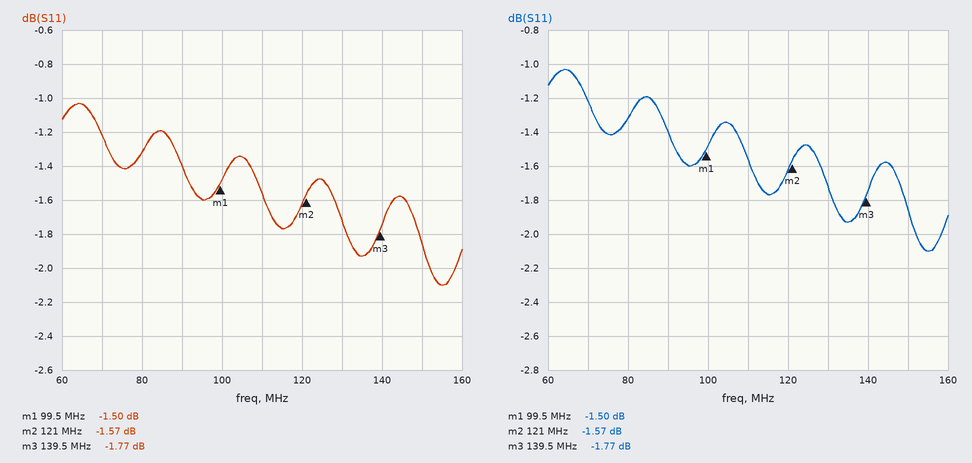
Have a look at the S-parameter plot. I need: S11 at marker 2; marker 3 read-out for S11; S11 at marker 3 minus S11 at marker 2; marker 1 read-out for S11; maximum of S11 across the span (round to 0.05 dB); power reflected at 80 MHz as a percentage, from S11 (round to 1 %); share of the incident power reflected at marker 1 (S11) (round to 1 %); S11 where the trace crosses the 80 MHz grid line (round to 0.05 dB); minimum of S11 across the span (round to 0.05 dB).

-1.57 dB
-1.77 dB
-0.20 dB
-1.50 dB
-1.05 dB
74 %
71 %
-1.30 dB
-2.10 dB
